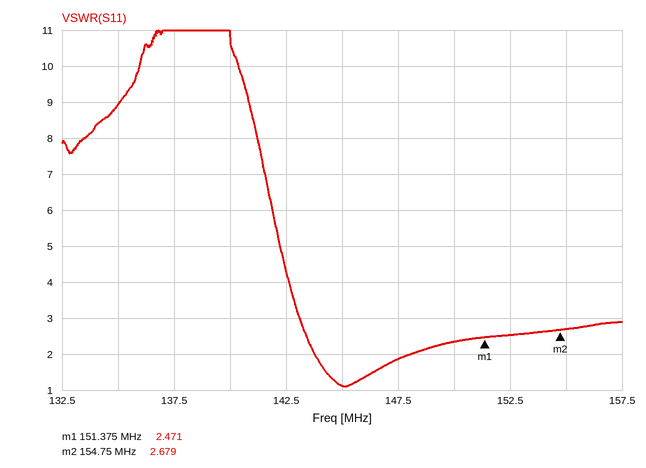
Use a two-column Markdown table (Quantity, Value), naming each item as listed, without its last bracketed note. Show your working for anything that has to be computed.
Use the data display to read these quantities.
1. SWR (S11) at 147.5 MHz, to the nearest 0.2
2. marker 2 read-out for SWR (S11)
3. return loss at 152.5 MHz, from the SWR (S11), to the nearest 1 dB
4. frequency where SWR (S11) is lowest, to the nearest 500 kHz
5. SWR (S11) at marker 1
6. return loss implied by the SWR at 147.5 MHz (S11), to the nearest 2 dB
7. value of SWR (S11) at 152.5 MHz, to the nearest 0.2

| Quantity | Value |
|---|---|
| SWR (S11) at 147.5 MHz, to the nearest 0.2 | 1.8 |
| marker 2 read-out for SWR | 2.679 |
| return loss at 152.5 MHz, from the SWR (S11), to the nearest 1 dB | −20 log10((2.6 − 1)/(2.6 + 1)) ≈ 7 dB |
| frequency where SWR (S11) is lowest, to the nearest 500 kHz | 145.0 MHz |
| SWR (S11) at marker 1 | 2.471 |
| return loss implied by the SWR at 147.5 MHz (S11), to the nearest 2 dB | −20 log10((1.8 − 1)/(1.8 + 1)) ≈ 10.9 dB, so 10 dB to the nearest 2 dB |
| value of SWR (S11) at 152.5 MHz, to the nearest 0.2 | 2.6 |
